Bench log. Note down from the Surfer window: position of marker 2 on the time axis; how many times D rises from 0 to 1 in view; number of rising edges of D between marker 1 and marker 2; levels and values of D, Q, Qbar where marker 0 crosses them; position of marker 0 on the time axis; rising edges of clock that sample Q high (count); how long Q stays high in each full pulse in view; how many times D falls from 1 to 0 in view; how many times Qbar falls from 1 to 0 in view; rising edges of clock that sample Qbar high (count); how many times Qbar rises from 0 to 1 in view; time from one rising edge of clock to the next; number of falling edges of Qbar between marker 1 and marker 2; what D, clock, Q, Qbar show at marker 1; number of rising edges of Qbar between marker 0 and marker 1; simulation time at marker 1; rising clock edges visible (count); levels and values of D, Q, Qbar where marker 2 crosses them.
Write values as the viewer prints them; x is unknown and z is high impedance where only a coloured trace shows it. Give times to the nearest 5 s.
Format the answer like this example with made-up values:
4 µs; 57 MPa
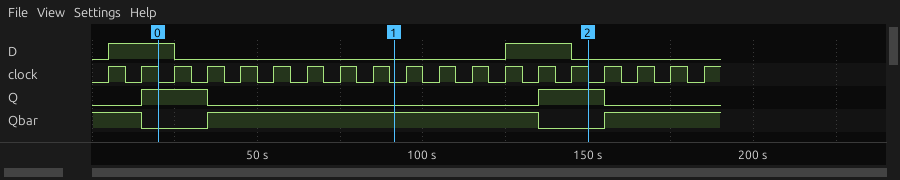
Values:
150 s; 2; 1; D=1, Q=1, Qbar=0; 20 s; 4; 20 s, 20 s; 2; 2; 15; 2; 10 s; 1; D=0, clock=0, Q=0, Qbar=1; 1; 90 s; 19; D=0, Q=1, Qbar=0
